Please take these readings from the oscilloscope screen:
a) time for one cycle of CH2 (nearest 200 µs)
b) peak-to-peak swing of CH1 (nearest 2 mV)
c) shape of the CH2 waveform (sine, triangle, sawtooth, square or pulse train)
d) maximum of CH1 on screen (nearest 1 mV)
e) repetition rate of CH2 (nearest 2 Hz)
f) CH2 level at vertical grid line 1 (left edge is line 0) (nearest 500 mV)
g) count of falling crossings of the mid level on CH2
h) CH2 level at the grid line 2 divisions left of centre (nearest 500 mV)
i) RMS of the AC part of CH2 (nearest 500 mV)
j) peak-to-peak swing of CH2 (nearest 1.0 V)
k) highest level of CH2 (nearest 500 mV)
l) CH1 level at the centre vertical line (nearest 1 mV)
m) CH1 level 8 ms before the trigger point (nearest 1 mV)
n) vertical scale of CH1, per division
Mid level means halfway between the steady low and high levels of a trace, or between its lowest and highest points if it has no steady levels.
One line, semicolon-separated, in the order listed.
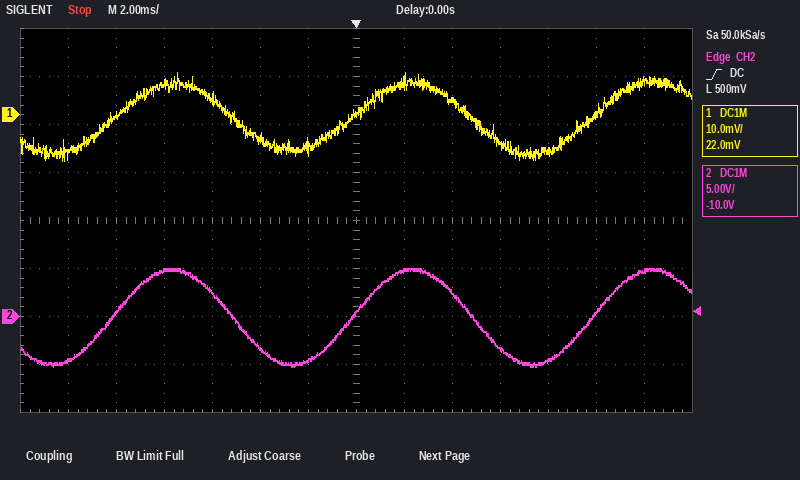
10.0 ms; 18 mV; sine; 9 mV; 100 Hz; -4.5 V; 2; -3.5 V; 3.5 V; 10.0 V; 5.0 V; 0 mV; 7 mV; 10 mV
